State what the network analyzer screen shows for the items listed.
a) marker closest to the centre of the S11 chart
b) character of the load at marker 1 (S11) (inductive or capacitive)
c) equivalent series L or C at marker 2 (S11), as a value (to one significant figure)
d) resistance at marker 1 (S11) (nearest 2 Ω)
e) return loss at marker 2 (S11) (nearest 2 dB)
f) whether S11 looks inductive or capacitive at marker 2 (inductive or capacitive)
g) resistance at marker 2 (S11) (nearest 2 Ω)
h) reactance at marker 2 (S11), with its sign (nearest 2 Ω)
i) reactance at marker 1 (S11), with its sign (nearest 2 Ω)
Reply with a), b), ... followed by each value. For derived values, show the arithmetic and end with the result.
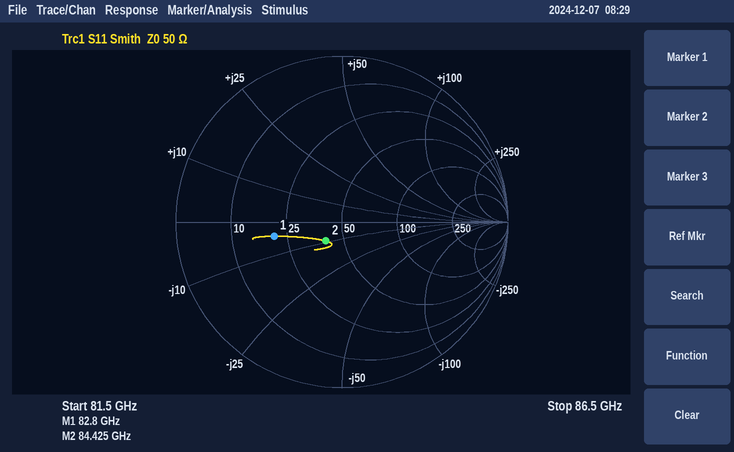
a) marker 2
b) capacitive
c) C = 1/(2π × 84.425 GHz × 10 Ω) ≈ 189 fF, so 200 fF to one significant figure
d) 20 Ω
e) 16 dB
f) capacitive
g) 40 Ω
h) -10 Ω
i) -4 Ω
